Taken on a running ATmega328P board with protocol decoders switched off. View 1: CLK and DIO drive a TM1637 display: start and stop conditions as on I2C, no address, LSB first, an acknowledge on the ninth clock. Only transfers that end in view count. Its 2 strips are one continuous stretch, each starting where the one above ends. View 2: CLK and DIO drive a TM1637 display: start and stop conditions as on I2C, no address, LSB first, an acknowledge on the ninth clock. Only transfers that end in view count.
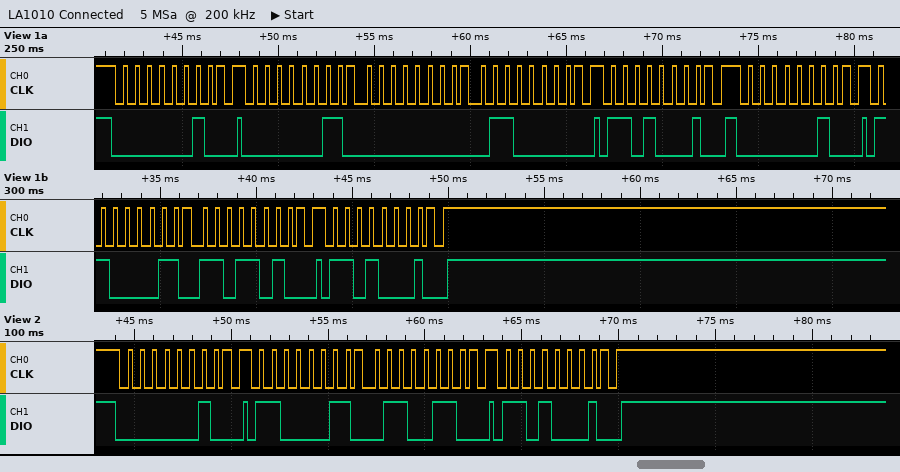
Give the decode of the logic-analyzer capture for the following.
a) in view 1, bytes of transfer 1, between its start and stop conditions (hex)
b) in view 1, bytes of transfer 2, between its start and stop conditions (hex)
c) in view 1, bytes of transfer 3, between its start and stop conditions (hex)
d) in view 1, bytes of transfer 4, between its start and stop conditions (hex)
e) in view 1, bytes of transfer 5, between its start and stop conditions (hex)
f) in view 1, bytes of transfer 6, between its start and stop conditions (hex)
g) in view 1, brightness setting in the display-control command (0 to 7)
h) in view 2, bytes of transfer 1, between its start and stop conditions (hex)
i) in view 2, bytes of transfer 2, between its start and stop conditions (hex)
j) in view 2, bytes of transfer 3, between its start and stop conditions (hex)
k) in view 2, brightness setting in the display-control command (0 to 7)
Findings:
40
C0 00 06
8B
40
C3 5B
8B
3
40
C3 66
8B
3
